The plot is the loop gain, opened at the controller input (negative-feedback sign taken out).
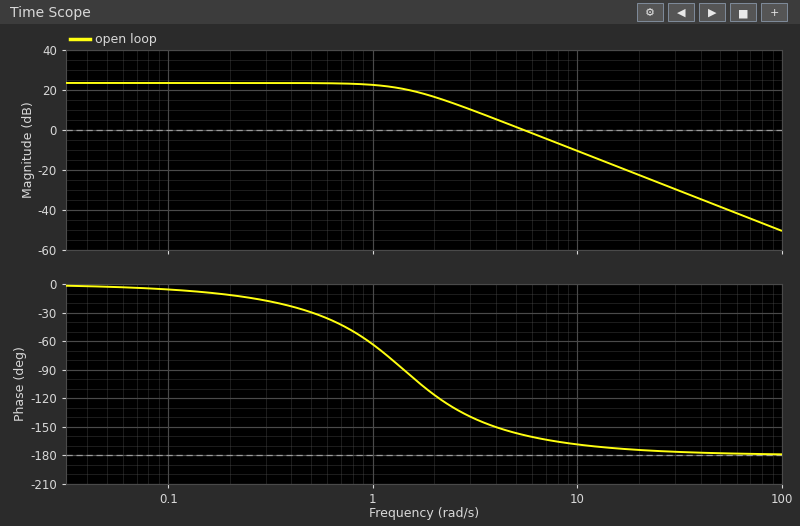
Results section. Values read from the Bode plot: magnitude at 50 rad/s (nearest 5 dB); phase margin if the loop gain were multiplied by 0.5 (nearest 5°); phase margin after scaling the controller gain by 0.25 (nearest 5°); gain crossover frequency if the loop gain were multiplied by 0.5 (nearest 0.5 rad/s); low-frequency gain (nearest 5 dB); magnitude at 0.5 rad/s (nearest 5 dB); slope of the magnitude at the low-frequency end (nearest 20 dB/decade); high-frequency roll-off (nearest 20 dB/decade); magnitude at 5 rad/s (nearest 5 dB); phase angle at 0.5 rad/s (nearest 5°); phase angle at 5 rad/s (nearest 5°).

-40 dB
30°
45°
4.0 rad/s
25 dB
25 dB
0 dB/decade
-40 dB/decade
0 dB
-30°
-155°
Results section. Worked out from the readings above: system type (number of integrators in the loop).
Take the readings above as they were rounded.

0
